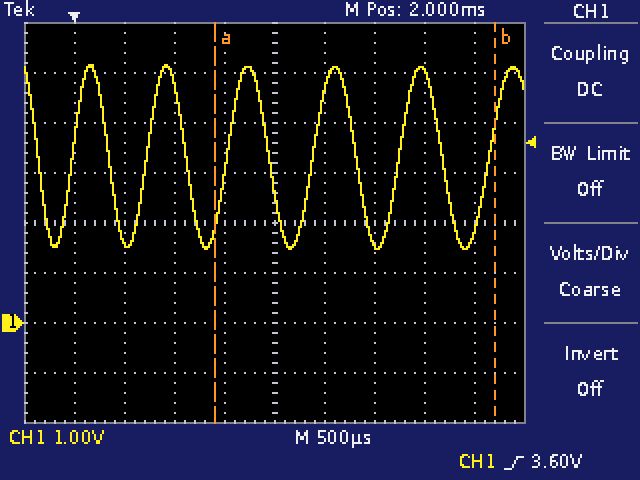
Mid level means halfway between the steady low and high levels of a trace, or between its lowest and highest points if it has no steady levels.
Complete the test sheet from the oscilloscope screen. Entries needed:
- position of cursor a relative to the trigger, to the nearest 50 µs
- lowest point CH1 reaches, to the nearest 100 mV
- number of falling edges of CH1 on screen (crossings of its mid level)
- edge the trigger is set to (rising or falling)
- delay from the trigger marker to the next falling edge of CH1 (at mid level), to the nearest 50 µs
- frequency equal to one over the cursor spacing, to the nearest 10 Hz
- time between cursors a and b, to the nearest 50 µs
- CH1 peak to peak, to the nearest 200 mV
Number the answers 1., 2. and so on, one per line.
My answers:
1. +1.40 ms
2. 1.5 V
3. 6
4. rising
5. 350 µs
6. 360 Hz
7. 2.80 ms
8. 3.6 V
